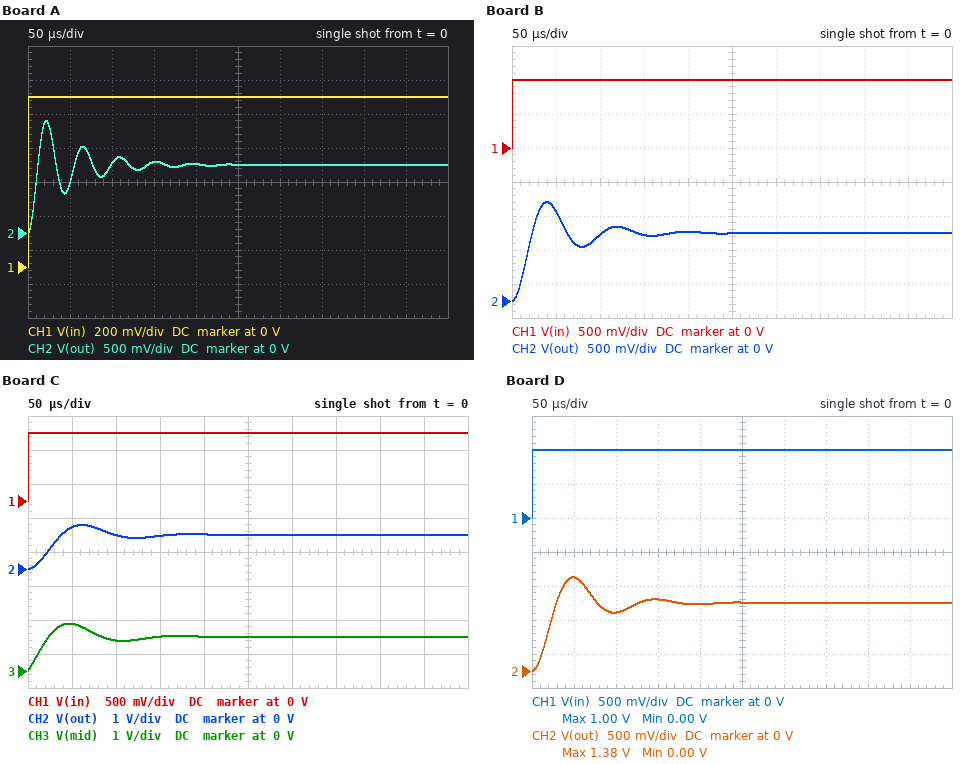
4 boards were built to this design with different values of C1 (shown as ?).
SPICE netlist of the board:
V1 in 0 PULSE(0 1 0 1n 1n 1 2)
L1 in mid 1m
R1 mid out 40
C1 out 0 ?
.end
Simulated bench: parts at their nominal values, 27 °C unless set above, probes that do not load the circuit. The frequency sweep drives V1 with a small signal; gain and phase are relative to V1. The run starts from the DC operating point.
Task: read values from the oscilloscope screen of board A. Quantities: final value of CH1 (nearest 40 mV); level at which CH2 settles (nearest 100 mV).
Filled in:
1.00 V
1.0 V
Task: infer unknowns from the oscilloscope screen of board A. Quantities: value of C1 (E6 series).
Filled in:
47 nF
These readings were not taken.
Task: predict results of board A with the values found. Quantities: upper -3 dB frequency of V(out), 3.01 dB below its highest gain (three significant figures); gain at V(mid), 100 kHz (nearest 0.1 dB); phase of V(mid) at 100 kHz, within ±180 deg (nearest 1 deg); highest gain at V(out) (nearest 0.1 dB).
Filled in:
25.8 kHz
-21.1 dB
-126 deg
11.3 dB
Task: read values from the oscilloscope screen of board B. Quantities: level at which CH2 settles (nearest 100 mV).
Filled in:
1.0 V
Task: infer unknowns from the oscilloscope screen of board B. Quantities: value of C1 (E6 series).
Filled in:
150 nF
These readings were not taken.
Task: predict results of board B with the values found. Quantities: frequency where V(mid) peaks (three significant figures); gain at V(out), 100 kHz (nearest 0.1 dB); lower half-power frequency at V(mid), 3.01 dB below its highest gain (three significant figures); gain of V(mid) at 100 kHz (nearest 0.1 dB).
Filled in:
12.3 kHz
-35.3 dB
8.70 kHz
-23.5 dB
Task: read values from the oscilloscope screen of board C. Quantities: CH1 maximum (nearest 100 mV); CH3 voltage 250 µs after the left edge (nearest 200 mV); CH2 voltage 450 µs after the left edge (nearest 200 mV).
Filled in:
1.0 V
1.0 V
1.0 V
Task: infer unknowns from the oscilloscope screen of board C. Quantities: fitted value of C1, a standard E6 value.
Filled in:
330 nF
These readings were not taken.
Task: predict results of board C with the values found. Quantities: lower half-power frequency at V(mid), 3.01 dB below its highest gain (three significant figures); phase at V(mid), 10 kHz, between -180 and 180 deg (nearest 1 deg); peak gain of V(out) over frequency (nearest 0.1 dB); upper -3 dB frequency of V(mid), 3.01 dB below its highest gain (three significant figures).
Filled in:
4.11 kHz
-70 deg
3.4 dB
11.1 kHz
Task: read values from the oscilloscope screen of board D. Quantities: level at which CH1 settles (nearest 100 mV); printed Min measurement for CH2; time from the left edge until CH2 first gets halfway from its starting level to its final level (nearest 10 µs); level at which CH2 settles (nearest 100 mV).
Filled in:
1.0 V
0.00 V
20 µs
1.0 V
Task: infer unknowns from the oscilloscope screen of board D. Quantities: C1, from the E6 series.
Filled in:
220 nF
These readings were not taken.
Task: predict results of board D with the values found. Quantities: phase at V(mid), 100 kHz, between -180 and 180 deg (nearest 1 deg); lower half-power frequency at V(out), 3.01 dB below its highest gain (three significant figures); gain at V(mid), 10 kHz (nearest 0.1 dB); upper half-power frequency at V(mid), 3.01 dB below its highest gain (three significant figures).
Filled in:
-97 deg
5.44 kHz
6.1 dB
13.1 kHz
